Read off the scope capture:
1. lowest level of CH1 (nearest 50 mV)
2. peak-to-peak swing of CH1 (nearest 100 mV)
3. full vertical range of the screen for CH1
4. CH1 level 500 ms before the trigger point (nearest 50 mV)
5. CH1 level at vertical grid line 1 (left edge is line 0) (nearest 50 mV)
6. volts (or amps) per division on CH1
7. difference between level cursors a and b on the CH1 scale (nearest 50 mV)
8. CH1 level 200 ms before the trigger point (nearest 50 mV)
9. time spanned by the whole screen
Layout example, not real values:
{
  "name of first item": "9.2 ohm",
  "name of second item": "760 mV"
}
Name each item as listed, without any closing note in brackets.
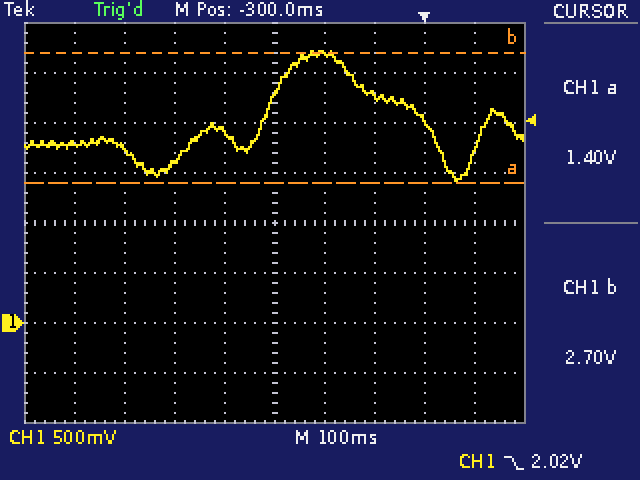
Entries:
{
  "lowest level of CH1": "1.40 V",
  "peak-to-peak swing of CH1": "1.30 V",
  "full vertical range of the screen for CH1": "4 V",
  "CH1 level 500 ms before the trigger point": "1.60 V",
  "CH1 level at vertical grid line 1 (left edge is line 0)": "1.80 V",
  "volts (or amps) per division on CH1": "500 mV",
  "difference between level cursors a and b on the CH1 scale": "1.30 V",
  "CH1 level 200 ms before the trigger point": "2.70 V",
  "time spanned by the whole screen": "1 s"
}
